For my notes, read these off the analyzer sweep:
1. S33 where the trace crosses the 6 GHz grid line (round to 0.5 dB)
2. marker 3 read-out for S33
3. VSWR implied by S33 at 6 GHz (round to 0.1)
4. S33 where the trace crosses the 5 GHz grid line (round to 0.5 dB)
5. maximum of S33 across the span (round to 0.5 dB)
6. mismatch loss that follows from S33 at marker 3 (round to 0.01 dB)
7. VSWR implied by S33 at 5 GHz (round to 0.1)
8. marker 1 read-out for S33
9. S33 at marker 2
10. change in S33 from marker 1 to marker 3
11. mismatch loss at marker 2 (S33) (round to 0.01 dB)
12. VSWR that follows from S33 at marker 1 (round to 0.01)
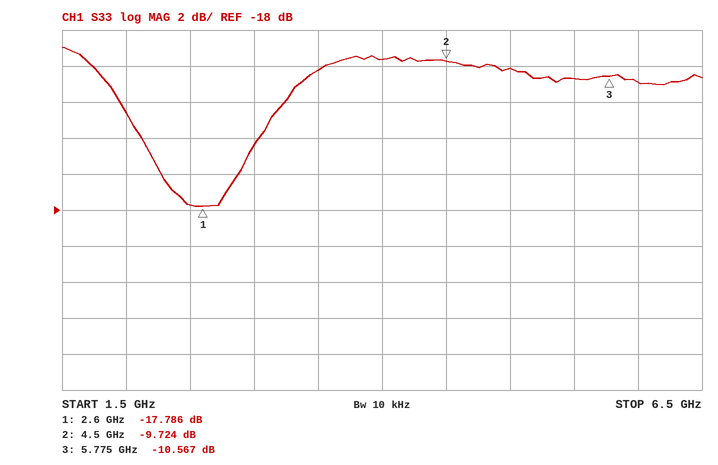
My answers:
-11.0 dB
-10.567 dB
1.8
-10.0 dB
-9.0 dB
0.40 dB
1.9
-17.786 dB
-9.724 dB
7.219 dB
0.49 dB
1.30
